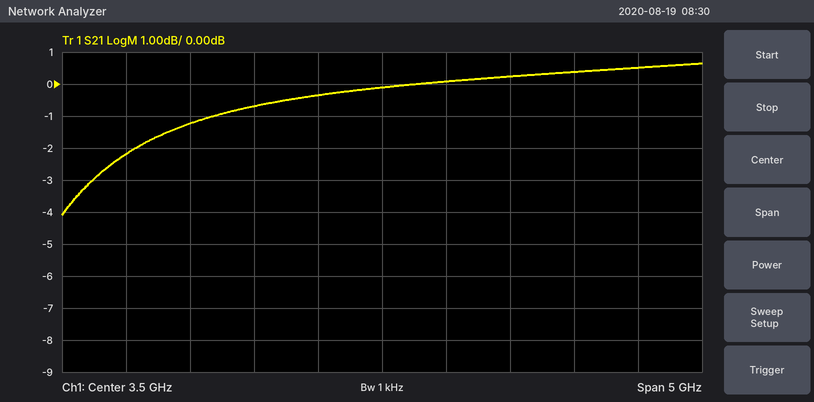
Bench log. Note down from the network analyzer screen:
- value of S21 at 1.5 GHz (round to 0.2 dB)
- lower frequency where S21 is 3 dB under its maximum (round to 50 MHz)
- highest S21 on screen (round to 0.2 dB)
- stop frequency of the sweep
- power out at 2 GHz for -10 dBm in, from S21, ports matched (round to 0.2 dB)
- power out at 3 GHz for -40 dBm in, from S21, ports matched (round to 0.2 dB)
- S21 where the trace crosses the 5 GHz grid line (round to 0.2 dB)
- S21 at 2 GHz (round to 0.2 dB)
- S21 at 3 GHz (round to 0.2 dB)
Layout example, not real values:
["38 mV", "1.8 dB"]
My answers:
["-2.2 dB", "1.45 GHz", "0.6 dB", "6 GHz", "-11.2 dBm", "-40.4 dBm", "0.4 dB", "-1.2 dB", "-0.4 dB"]
